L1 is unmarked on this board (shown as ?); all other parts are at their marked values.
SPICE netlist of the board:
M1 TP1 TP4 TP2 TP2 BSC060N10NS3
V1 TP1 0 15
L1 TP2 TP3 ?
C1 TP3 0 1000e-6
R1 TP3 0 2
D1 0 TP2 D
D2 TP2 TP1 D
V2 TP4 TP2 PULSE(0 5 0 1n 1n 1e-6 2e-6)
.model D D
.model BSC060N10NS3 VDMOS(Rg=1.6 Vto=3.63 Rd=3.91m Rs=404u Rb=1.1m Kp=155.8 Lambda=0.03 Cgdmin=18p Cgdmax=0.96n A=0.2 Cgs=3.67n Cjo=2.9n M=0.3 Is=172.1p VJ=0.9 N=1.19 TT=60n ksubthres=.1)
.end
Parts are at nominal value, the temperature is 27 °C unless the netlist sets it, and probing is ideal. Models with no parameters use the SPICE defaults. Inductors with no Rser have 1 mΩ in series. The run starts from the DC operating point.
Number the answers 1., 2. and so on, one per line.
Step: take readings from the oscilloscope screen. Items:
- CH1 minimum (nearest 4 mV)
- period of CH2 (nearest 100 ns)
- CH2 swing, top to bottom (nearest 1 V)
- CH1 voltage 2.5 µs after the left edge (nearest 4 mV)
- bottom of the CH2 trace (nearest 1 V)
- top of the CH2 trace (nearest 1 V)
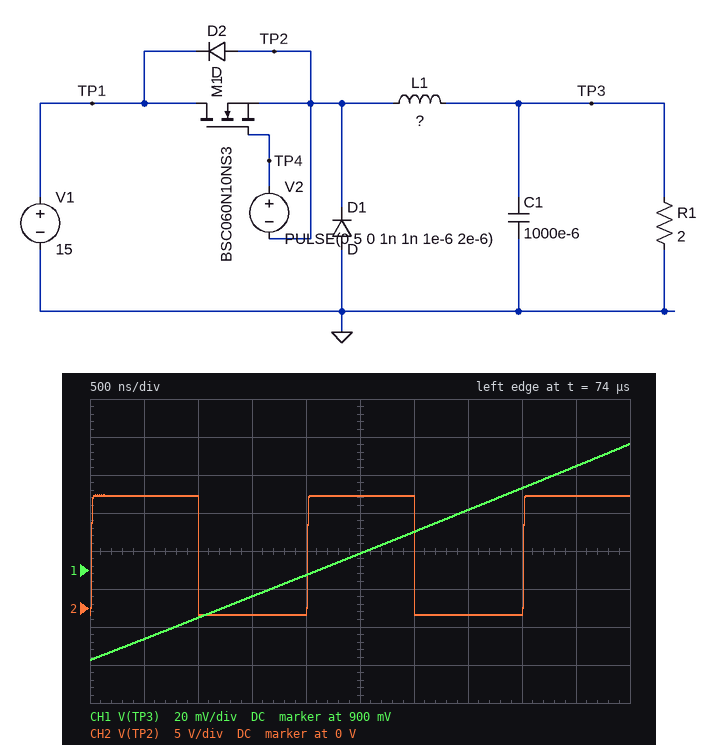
1. 852 mV
2. 2.0 µs
3. 16 V
4. 908 mV
5. -1 V
6. 15 V
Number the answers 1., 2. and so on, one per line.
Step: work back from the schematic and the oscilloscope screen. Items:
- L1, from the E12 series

1. 22 µH
